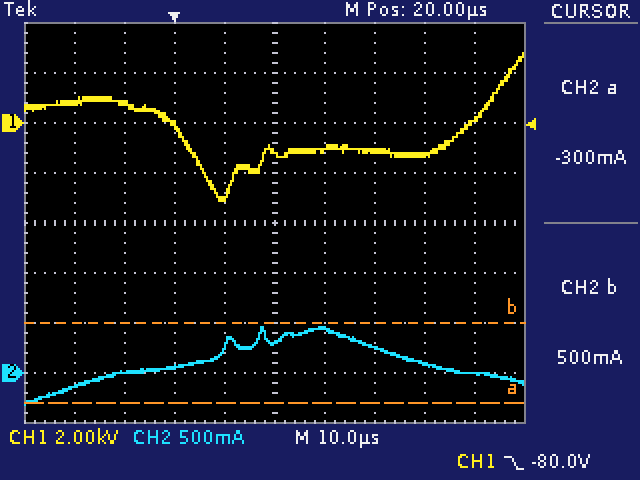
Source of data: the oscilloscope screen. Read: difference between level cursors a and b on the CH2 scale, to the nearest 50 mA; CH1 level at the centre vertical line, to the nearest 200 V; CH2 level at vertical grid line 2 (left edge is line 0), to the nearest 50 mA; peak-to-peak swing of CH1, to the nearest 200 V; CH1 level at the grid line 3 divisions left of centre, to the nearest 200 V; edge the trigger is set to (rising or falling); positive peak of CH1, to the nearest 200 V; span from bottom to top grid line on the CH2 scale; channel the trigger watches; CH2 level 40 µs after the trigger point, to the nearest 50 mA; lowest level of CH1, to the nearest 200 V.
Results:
800 mA
-1.2 kV
0 mA
6.0 kV
800 V
falling
2.8 kV
4 A
CH1
250 mA
-3.2 kV
